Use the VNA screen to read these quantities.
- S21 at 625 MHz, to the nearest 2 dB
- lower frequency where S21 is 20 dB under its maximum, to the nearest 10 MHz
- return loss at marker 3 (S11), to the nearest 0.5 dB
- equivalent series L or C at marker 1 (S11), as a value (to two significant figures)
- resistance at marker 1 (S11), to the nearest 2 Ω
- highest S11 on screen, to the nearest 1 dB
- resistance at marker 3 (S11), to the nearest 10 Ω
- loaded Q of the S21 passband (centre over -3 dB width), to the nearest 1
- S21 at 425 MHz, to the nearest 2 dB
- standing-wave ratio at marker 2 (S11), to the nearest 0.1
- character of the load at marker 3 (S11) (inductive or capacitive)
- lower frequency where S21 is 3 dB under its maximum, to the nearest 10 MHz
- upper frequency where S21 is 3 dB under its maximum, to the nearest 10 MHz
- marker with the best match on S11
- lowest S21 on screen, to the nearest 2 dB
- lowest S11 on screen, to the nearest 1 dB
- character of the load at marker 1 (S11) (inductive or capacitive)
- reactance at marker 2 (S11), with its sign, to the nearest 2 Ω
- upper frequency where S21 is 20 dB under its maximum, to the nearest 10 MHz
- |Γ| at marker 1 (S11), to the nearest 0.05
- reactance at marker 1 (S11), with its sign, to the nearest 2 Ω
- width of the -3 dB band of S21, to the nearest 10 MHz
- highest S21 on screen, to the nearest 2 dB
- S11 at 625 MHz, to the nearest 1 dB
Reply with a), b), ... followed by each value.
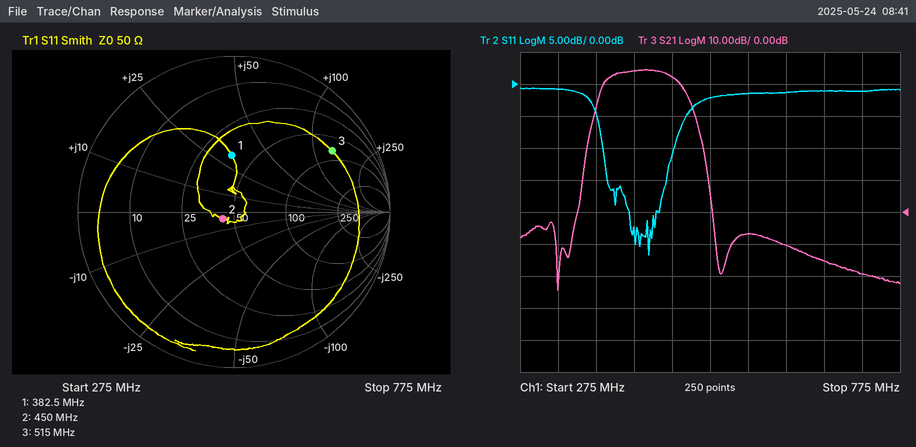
a) -10 dB
b) 370 MHz
c) 2.5 dB
d) 13 nH
e) 38 Ω
f) -1 dB
g) 80 Ω
h) 5
i) 44 dB
j) 1.2
k) inductive
l) 390 MHz
m) 480 MHz
n) marker 2
o) -24 dB
p) -27 dB
q) inductive
r) -4 Ω
s) 510 MHz
t) 0.35
u) +32 Ω
v) 90 MHz
w) 44 dB
x) -1 dB
